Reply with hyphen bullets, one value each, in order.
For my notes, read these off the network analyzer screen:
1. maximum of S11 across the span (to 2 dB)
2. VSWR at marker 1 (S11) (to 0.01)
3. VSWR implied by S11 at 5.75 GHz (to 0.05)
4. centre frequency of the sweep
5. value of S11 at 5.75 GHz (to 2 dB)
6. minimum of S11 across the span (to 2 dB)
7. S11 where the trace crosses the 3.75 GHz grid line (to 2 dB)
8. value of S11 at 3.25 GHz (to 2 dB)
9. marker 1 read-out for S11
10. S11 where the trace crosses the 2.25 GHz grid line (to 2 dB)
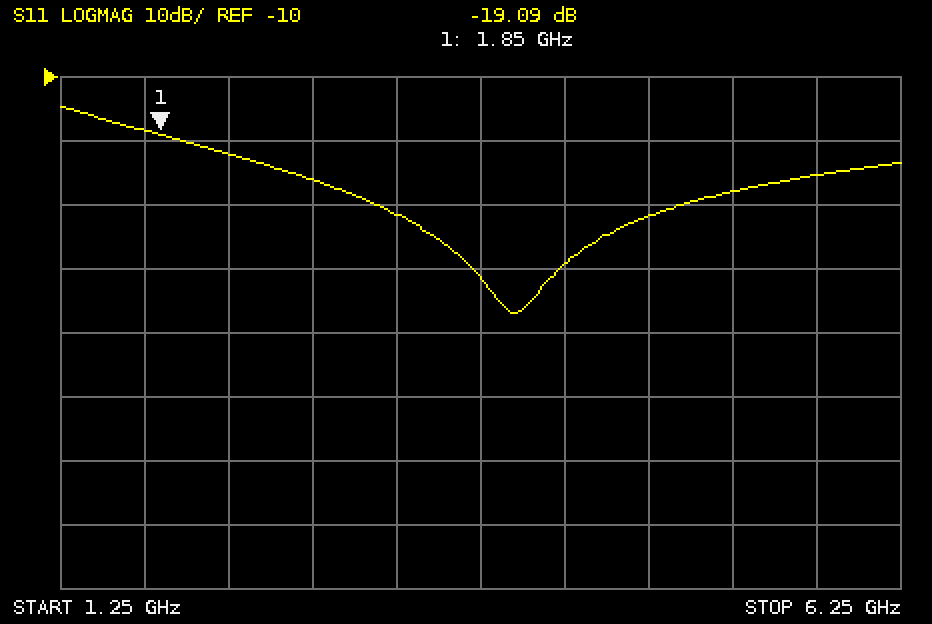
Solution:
- -14 dB
- 1.25
- 1.10
- 3.75 GHz
- -26 dB
- -46 dB
- -42 dB
- -32 dB
- -19.09 dB
- -22 dB
